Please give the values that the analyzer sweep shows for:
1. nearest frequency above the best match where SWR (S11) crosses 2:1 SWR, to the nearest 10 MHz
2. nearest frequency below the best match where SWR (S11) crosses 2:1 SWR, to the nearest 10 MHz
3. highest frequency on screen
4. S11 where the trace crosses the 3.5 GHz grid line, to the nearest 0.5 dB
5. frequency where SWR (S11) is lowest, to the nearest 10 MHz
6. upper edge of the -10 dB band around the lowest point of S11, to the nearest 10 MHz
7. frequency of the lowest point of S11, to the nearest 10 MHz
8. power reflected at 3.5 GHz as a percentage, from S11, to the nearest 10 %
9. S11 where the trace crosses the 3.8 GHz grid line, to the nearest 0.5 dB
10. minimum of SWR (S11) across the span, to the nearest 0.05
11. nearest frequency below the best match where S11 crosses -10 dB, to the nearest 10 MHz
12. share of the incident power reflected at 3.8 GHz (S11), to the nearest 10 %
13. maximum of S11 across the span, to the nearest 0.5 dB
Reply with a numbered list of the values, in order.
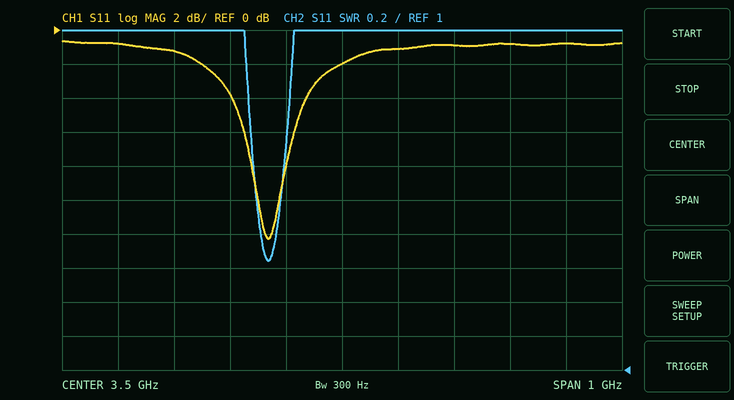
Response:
1. 3.39 GHz
2. 3.35 GHz
3. 4 GHz
4. -2.0 dB
5. 3.37 GHz
6. 3.39 GHz
7. 3.37 GHz
8. 60 %
9. -1.0 dB
10. 1.65
11. 3.35 GHz
12. 80 %
13. -0.5 dB
